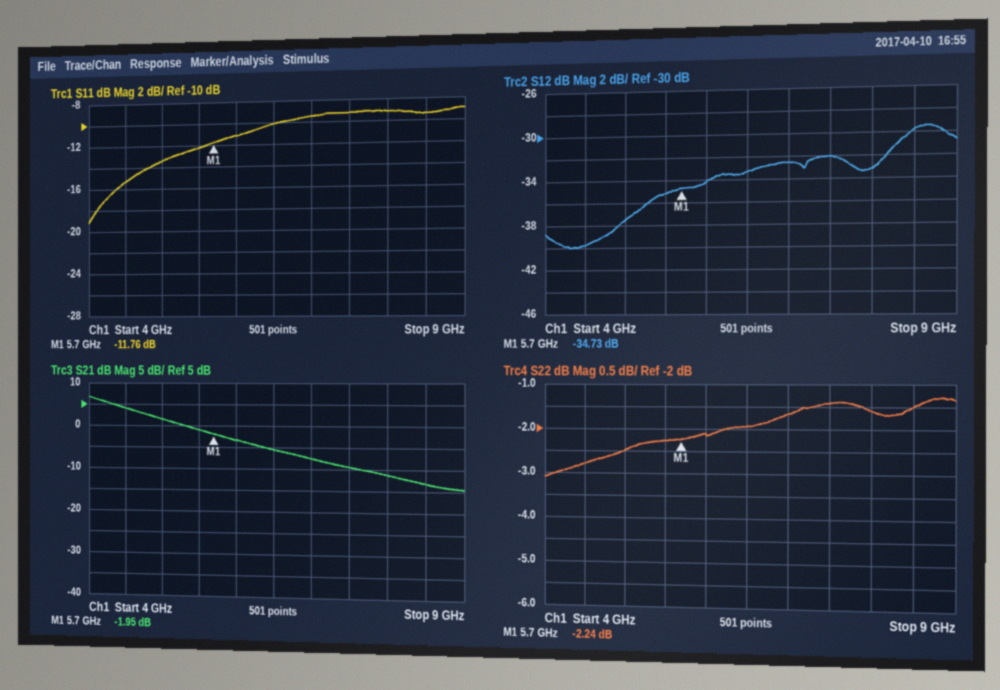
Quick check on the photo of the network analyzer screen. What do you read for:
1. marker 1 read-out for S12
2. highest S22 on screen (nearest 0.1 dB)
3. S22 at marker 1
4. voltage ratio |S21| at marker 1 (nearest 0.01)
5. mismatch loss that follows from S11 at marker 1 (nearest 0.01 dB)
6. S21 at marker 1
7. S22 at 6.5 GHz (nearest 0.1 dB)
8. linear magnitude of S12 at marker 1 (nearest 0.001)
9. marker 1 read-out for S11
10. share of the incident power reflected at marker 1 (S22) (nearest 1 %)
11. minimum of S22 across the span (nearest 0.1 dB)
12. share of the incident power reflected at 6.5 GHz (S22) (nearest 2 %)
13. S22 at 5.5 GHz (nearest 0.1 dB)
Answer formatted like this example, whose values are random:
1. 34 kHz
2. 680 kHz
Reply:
1. -34.73 dB
2. -1.3 dB
3. -2.24 dB
4. 0.80
5. 0.30 dB
6. -1.95 dB
7. -1.9 dB
8. 0.018
9. -11.76 dB
10. 60 %
11. -3.1 dB
12. 64 %
13. -2.3 dB
